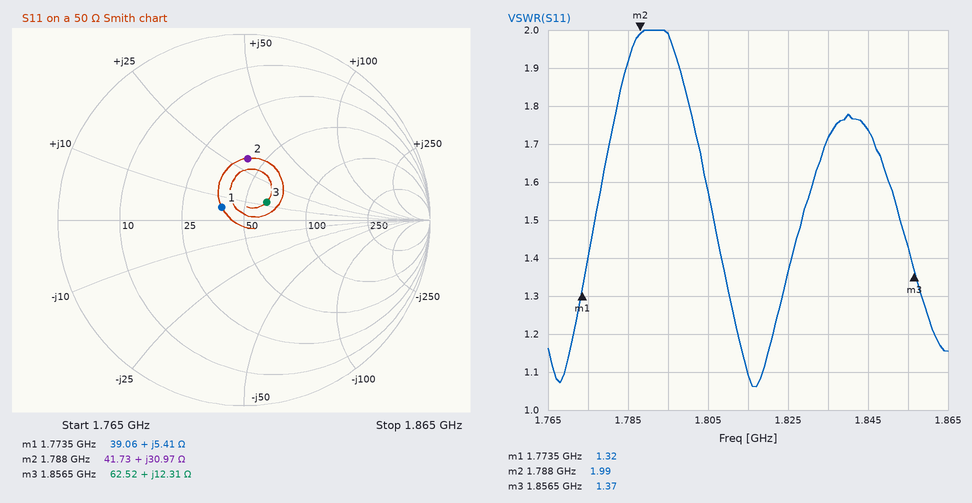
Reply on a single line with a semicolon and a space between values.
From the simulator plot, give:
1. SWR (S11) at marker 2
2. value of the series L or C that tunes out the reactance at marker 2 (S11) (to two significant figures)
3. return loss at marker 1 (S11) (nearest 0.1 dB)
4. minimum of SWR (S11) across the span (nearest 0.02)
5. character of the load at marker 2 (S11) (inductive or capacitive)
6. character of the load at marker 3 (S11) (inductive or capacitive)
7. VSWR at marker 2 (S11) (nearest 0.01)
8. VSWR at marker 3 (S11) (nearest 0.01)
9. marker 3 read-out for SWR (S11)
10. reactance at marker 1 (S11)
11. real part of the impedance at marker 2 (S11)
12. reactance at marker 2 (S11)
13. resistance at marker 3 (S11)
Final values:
1.99; 2.9 pF; 17.3 dB; 1.06; inductive; inductive; 1.99; 1.37; 1.37; +5.41 Ω; 41.73 Ω; +30.97 Ω; 62.52 Ω
